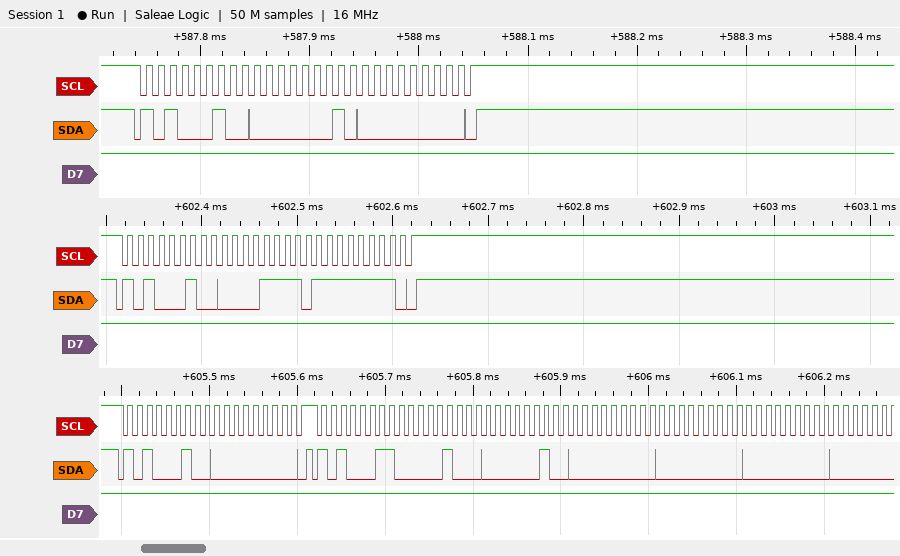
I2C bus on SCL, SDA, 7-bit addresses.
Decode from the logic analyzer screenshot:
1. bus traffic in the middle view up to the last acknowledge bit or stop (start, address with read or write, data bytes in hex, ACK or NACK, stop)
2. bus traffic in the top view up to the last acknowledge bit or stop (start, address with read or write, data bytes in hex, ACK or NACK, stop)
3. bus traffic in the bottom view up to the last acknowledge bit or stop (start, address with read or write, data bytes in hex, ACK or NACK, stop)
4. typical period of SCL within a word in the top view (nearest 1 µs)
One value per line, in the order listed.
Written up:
start, address 51 write ACK, 0F ACK, FF ACK, stop
start, address 51 write ACK, 01 ACK, 00 ACK, stop
start, address 51 write ACK, 00 ACK, stop, start, address 51 read ACK, 08 ACK, 04 ACK, 00 ACK, 00 ACK, 00 ACK
11 µs
